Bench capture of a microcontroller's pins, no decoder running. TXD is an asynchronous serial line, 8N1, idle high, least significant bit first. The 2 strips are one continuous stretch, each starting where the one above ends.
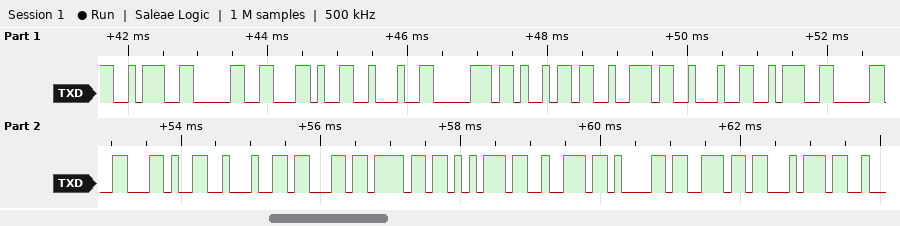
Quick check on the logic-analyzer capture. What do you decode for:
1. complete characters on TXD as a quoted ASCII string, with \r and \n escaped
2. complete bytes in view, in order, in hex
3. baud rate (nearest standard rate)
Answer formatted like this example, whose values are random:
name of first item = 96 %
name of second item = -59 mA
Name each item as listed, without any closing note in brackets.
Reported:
complete characters on TXD as a quoted ASCII string, with \r and \n escaped = ":0,\"pir\":0,\"courant"
complete bytes in view, in order, in hex = 3A 30 2C 22 70 69 72 22 3A 30 2C 22 63 6F 75 72 61 6E 74
baud rate = 9600 baud
